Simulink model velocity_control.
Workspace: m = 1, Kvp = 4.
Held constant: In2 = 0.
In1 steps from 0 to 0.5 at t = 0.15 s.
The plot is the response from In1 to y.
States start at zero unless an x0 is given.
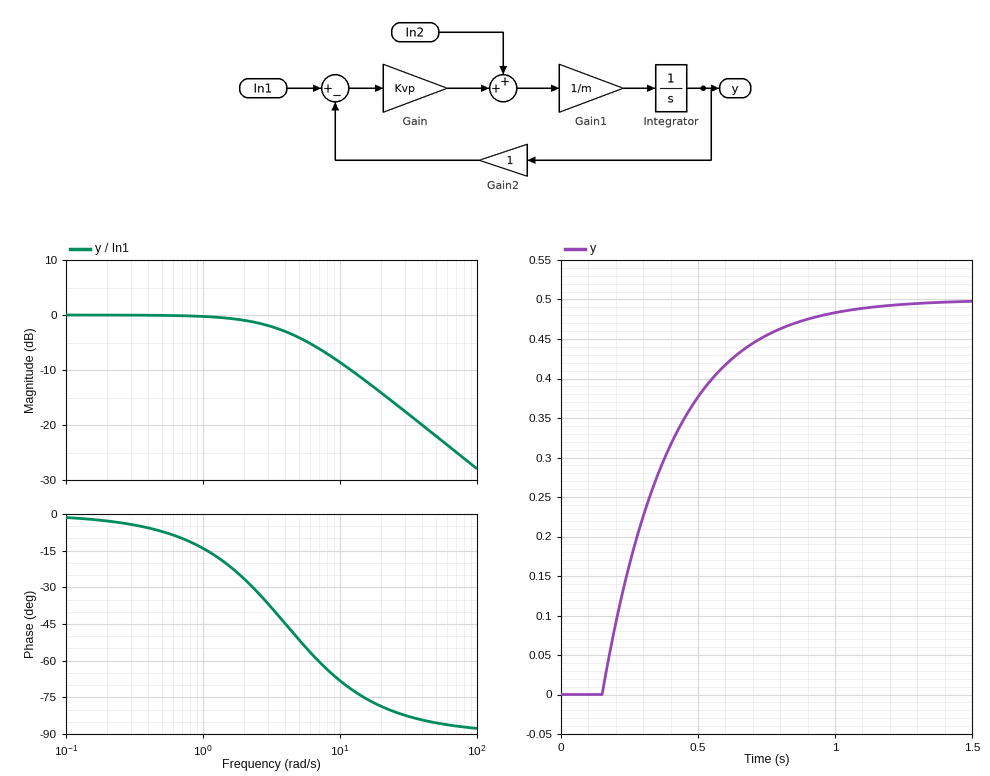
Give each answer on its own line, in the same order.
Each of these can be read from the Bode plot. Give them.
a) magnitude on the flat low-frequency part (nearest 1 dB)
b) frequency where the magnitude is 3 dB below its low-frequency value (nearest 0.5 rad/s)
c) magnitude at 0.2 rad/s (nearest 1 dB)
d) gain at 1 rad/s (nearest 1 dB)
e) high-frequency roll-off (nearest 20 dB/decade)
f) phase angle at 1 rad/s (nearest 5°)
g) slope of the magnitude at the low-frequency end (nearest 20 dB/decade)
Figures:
0 dB
4.0 rad/s
0 dB
0 dB
-20 dB/decade
-15°
0 dB/decade
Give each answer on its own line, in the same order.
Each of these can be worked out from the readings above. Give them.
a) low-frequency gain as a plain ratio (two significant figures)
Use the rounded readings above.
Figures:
1.0
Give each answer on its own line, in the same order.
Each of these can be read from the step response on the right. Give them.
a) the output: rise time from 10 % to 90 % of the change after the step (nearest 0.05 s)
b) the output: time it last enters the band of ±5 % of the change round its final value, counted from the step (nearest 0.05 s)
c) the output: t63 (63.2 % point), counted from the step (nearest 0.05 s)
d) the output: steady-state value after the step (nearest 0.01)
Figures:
0.55 s
0.75 s
0.25 s
0.50
